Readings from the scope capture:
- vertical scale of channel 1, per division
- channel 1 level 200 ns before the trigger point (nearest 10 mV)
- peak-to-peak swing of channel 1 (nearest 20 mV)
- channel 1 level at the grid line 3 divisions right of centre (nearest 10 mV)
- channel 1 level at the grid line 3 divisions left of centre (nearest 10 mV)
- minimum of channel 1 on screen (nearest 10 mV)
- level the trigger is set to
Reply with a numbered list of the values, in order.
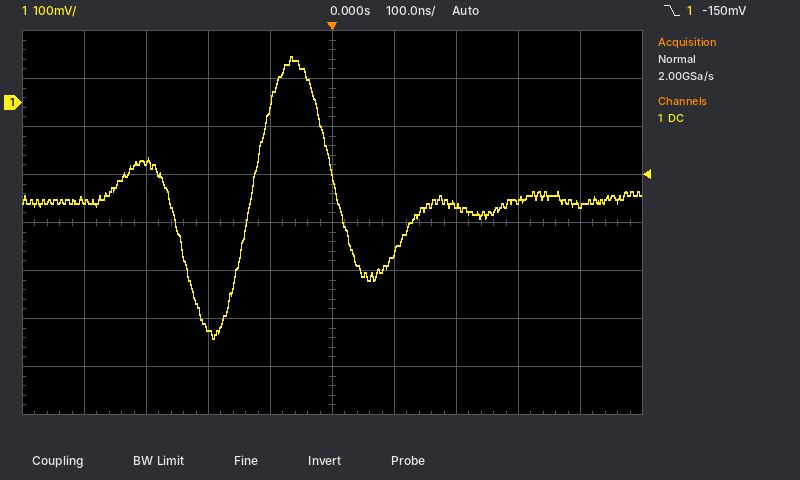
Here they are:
1. 100 mV
2. -470 mV
3. 580 mV
4. -200 mV
5. -120 mV
6. -490 mV
7. -150 mV
